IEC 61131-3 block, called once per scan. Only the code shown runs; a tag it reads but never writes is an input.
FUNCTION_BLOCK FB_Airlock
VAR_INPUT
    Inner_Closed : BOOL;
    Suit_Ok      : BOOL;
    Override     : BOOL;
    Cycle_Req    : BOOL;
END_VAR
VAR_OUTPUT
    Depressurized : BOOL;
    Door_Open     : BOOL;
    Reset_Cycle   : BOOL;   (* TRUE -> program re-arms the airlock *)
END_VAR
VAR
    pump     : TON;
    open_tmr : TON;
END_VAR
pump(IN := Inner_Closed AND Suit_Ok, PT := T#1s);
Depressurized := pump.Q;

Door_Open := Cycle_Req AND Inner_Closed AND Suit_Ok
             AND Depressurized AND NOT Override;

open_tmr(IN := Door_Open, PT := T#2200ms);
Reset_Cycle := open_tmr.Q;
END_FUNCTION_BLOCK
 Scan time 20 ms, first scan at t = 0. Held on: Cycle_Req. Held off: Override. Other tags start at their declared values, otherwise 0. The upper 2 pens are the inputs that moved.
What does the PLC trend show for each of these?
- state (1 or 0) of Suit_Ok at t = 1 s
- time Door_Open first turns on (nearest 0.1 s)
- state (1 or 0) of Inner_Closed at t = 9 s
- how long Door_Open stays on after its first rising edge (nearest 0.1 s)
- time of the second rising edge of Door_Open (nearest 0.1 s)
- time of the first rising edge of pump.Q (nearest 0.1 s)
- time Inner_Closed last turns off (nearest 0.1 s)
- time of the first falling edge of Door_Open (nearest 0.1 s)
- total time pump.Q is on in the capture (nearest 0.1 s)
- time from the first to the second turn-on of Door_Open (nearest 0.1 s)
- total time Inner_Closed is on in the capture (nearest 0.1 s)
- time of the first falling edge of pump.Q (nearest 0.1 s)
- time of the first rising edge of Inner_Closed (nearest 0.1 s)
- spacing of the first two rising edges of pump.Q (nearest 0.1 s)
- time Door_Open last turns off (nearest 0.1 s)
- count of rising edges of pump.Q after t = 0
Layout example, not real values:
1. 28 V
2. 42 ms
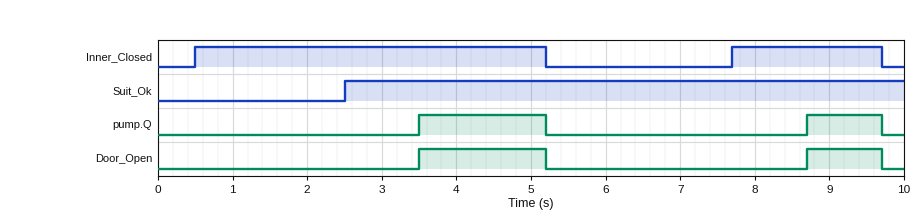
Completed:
1. 0
2. 3.5 s
3. 1
4. 1.7 s
5. 8.7 s
6. 3.5 s
7. 9.7 s
8. 5.2 s
9. 2.7 s
10. 5.2 s
11. 6.7 s
12. 5.2 s
13. 0.5 s
14. 5.2 s
15. 9.7 s
16. 2
